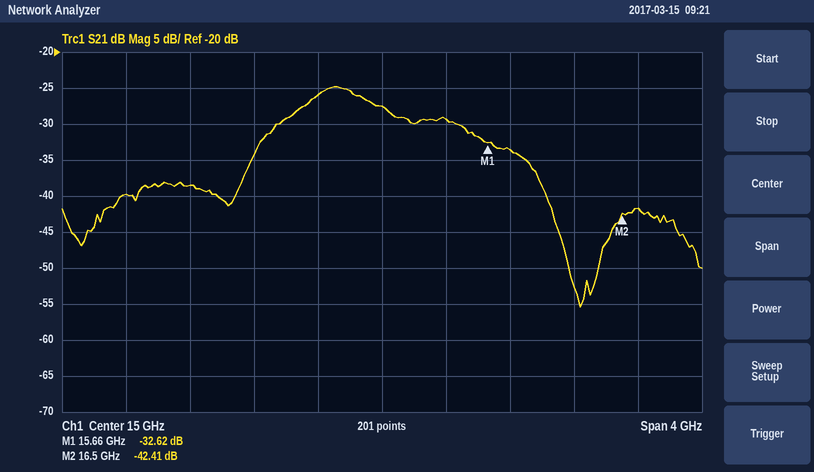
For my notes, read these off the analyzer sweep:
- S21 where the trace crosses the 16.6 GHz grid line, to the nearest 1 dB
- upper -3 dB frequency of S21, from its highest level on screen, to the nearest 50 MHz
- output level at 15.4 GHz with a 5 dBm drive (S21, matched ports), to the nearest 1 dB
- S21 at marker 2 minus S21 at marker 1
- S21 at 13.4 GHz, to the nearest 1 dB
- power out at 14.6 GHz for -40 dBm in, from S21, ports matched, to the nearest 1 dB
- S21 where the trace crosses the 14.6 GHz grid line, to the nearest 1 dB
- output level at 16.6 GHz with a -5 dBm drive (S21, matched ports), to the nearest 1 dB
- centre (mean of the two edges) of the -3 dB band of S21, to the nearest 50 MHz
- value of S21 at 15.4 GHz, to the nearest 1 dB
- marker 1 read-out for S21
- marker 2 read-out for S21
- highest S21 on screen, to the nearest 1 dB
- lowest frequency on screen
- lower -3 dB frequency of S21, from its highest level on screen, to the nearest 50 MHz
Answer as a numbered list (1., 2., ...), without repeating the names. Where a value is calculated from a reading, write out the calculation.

1. -42 dB
2. 15.00 GHz
3. 5 dBm + (-29 dB) = -24 dBm
4. -42.41 − (-32.62) = -9.79 dB
5. -40 dB
6. -40 dBm + (-26 dB) = -66 dBm
7. -26 dB
8. -5 dBm + (-42 dB) = -47 dBm
9. 14.75 GHz
10. -29 dB
11. -32.62 dB
12. -42.41 dB
13. -25 dB
14. 13 GHz
15. 14.50 GHz
